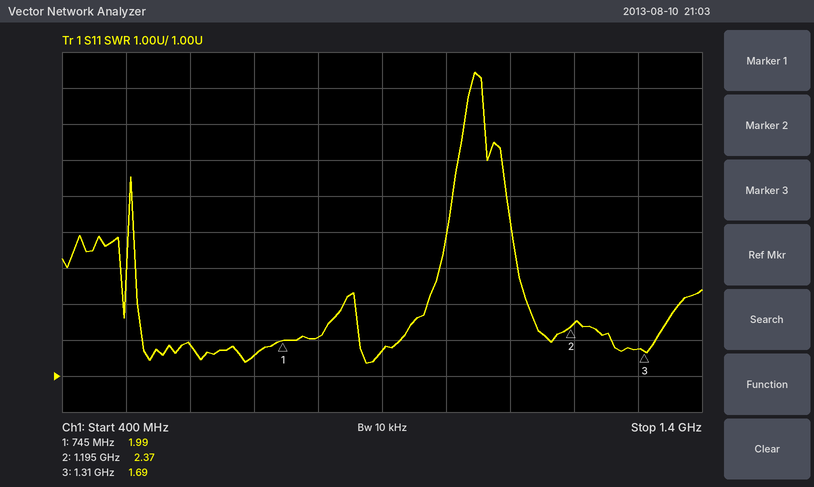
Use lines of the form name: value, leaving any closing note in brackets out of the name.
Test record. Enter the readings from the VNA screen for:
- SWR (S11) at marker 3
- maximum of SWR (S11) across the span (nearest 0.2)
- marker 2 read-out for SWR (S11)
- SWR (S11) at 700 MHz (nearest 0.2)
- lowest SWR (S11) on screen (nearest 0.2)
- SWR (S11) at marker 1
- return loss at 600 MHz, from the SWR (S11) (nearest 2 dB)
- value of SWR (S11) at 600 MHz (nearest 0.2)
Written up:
SWR (S11) at marker 3: 1.69
maximum of SWR (S11) across the span: 9.4
marker 2 read-out for SWR: 2.37
SWR (S11) at 700 MHz: 1.6
lowest SWR (S11) on screen: 1.4
SWR (S11) at marker 1: 1.99
return loss at 600 MHz, from the SWR (S11): 10 dB
value of SWR (S11) at 600 MHz: 1.8
